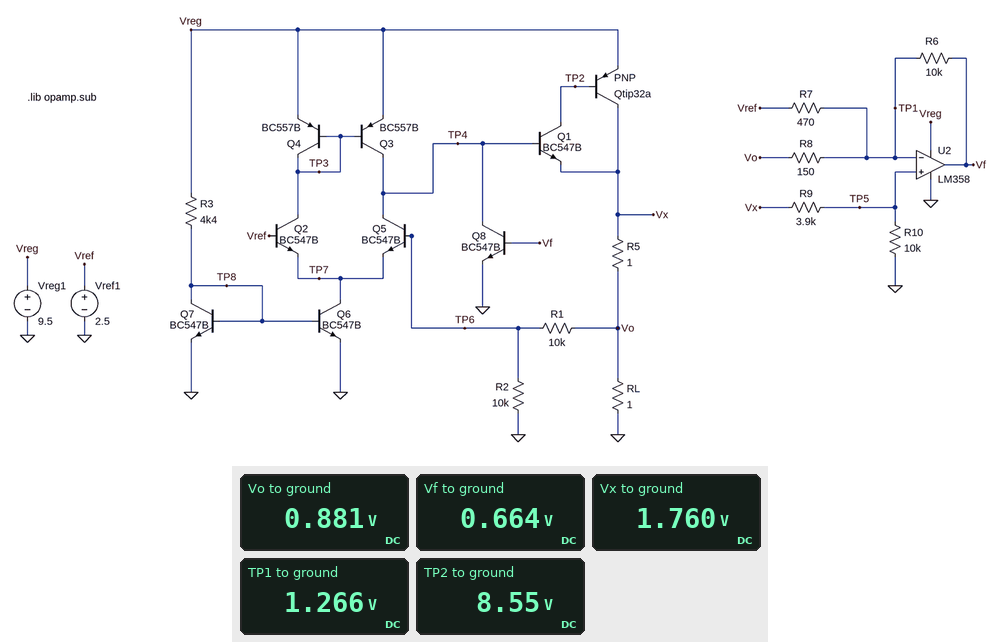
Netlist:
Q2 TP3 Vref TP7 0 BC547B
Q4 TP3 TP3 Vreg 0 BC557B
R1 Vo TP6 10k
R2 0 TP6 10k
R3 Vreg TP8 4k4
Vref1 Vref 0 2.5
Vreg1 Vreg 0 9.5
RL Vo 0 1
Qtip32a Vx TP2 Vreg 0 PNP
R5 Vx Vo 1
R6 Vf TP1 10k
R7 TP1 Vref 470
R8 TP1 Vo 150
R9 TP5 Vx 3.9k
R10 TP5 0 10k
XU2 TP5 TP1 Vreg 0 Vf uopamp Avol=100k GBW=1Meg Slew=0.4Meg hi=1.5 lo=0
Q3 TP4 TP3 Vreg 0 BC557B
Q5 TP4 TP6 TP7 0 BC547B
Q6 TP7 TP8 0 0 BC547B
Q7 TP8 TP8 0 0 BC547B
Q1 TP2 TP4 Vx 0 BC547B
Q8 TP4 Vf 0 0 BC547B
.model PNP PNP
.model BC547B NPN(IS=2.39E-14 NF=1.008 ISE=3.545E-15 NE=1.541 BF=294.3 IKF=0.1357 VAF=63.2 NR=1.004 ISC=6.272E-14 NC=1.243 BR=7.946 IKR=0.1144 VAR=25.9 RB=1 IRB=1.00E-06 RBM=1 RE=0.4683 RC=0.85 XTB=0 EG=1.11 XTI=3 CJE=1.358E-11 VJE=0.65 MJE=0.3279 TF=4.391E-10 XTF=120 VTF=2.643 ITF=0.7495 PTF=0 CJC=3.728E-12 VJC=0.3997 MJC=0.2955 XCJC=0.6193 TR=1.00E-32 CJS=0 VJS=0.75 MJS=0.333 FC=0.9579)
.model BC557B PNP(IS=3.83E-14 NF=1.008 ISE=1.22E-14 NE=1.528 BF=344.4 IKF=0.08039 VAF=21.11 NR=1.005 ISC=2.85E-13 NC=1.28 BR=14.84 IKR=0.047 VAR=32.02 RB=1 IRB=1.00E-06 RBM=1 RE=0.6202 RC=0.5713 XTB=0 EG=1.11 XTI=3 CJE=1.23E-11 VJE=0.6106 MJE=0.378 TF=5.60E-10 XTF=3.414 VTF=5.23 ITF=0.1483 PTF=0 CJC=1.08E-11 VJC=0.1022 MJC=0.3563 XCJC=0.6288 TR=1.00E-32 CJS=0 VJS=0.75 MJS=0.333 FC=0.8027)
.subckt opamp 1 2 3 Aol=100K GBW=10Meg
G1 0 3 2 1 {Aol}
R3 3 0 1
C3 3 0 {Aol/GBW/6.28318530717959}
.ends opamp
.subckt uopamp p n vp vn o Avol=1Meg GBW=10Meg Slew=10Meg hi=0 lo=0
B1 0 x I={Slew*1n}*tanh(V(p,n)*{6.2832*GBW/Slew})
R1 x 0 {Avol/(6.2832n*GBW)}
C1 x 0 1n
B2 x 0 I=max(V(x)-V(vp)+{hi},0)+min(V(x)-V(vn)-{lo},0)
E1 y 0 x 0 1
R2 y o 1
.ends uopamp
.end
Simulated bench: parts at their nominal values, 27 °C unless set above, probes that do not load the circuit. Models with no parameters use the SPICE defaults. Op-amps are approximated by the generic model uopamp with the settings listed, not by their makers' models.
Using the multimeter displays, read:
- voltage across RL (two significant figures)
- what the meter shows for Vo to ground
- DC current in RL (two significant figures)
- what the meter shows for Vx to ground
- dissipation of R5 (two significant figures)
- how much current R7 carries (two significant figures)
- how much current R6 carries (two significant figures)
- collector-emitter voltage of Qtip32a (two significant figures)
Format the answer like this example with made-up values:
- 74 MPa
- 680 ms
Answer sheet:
- 880 mV
- 0.881 V
- 880 mA
- 1.760 V
- 770 mW
- 2.6 mA
- 60 µA
- -7.7 V
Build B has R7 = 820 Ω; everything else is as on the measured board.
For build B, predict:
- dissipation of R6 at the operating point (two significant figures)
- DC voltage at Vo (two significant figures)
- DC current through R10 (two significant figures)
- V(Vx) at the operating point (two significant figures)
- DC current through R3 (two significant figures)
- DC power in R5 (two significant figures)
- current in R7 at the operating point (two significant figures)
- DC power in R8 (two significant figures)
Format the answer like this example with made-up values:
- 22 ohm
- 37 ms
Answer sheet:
- 7.1 µW
- 650 mV
- 93 µA
- 1.3 V
- 2.0 mA
- 420 mW
- 1.9 mA
- 530 µW
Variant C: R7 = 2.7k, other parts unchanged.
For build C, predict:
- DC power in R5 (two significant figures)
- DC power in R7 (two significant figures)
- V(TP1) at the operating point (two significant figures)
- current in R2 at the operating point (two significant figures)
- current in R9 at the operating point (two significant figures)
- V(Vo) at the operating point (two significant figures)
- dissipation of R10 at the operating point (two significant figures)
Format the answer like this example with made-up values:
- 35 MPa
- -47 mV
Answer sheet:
- 76 mW
- 1.6 mW
- 400 mV
- 14 µA
- 40 µA
- 280 mV
- 16 µW
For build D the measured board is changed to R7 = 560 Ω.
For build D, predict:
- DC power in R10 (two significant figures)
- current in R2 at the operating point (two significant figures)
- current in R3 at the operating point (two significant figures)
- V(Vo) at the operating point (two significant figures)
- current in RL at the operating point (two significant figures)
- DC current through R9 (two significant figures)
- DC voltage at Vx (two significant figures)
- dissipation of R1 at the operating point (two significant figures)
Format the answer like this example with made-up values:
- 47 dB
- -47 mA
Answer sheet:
- 130 µW
- 40 µA
- 2.0 mA
- 810 mV
- 810 mA
- 120 µA
- 1.6 V
- 16 µW
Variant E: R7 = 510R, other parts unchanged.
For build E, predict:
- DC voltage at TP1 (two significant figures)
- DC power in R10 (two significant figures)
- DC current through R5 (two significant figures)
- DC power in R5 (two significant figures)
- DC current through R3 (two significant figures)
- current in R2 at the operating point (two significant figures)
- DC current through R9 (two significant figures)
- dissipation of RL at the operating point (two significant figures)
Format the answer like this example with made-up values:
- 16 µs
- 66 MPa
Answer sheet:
- 1.2 V
- 150 µW
- 840 mA
- 710 mW
- 2.0 mA
- 42 µA
- 120 µA
- 720 mW
